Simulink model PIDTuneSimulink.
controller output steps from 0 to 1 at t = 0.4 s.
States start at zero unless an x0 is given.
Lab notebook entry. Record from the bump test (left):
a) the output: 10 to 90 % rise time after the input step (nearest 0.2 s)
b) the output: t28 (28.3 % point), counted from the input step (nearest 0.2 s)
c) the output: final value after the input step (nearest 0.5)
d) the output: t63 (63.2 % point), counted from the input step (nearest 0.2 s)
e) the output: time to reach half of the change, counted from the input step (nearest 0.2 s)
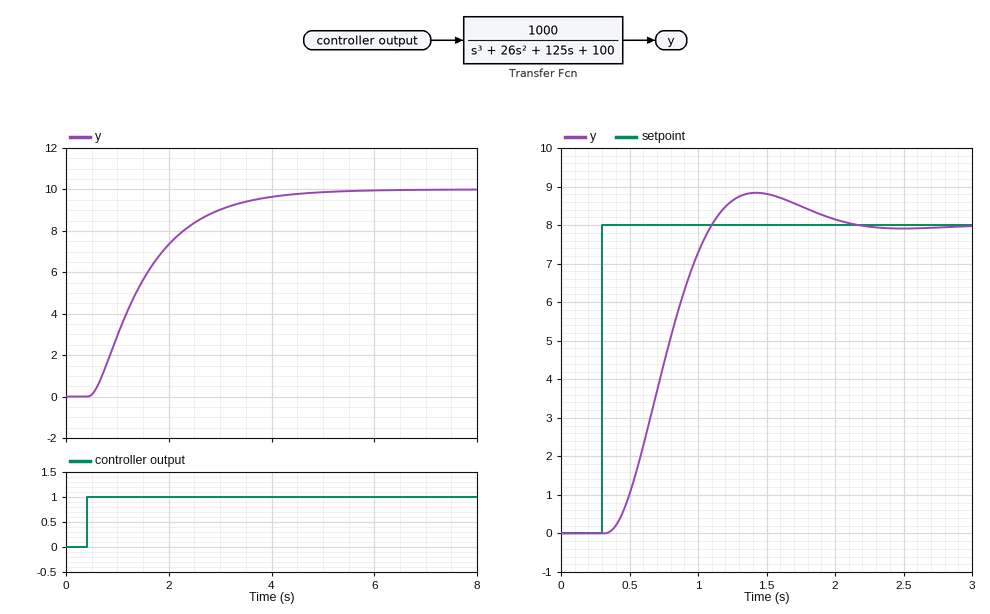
2.2 s
0.6 s
10.0
1.2 s
1.0 s
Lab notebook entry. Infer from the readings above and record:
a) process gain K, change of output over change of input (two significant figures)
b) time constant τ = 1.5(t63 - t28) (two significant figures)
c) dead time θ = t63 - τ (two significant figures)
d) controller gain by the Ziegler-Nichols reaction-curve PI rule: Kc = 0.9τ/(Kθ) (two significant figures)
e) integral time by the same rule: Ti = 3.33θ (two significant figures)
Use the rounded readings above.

10
0.90 s
0.30 s
0.27
1.00 s
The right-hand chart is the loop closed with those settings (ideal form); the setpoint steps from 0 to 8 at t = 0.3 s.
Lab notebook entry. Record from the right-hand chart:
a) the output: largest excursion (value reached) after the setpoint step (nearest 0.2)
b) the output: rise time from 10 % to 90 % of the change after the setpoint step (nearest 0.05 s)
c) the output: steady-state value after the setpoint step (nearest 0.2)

8.8
0.50 s
8.0
